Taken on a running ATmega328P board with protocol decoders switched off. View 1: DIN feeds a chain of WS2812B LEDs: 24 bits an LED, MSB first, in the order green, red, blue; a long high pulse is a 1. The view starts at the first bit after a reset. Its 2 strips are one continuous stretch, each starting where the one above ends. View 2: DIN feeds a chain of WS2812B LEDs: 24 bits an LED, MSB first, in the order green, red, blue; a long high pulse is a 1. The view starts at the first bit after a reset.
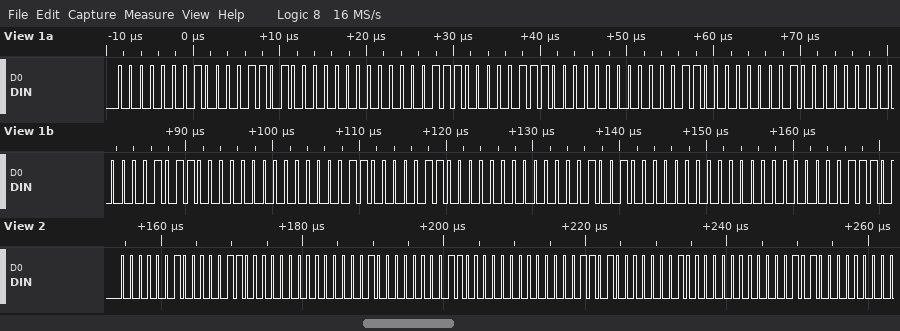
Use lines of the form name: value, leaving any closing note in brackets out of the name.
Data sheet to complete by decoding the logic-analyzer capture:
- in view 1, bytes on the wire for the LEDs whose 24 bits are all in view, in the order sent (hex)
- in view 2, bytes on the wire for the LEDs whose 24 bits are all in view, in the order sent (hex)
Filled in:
in view 1, bytes on the wire for the LEDs whose 24 bits are all in view, in the order sent: 01 0D 00 07 07 00 0C 02 00 0B 00 03 06 00 09 00 00 0E
in view 2, bytes on the wire for the LEDs whose 24 bits are all in view, in the order sent: 02 0C 00 08 06 00 0D 01 00
